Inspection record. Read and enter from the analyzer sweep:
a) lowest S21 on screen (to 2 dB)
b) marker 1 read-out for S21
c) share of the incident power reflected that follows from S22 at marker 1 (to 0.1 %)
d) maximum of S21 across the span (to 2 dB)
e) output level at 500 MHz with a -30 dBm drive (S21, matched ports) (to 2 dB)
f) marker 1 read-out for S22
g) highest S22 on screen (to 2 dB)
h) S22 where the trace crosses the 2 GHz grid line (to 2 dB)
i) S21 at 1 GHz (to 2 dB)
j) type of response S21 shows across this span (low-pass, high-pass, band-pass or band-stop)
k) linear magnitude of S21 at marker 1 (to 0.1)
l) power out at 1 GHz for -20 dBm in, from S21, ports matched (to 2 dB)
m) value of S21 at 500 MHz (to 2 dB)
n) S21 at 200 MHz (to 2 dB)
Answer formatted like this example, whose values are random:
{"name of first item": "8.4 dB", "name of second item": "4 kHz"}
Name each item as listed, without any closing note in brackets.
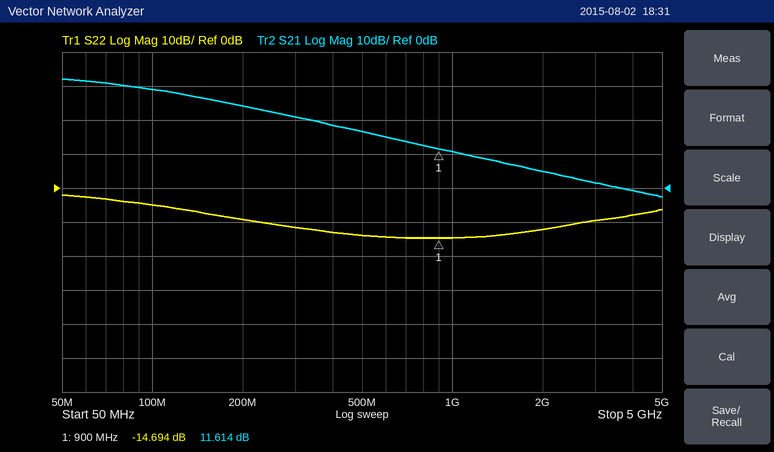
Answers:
{"lowest S21 on screen": "-2 dB", "marker 1 read-out for S21": "11.614 dB", "share of the incident power reflected that follows from S22 at marker 1": "3.4 %", "maximum of S21 across the span": "32 dB", "output level at 500 MHz with a -30 dBm drive (S21, matched ports)": "-14 dBm", "marker 1 read-out for S22": "-14.694 dB", "highest S22 on screen": "-2 dB", "S22 where the trace crosses the 2 GHz grid line": "-12 dB", "S21 at 1 GHz": "10 dB", "type of response S21 shows across this span": "low-pass", "linear magnitude of S21 at marker 1": "3.8", "power out at 1 GHz for -20 dBm in, from S21, ports matched": "-10 dBm", "value of S21 at 500 MHz": "16 dB", "S21 at 200 MHz": "24 dB"}
